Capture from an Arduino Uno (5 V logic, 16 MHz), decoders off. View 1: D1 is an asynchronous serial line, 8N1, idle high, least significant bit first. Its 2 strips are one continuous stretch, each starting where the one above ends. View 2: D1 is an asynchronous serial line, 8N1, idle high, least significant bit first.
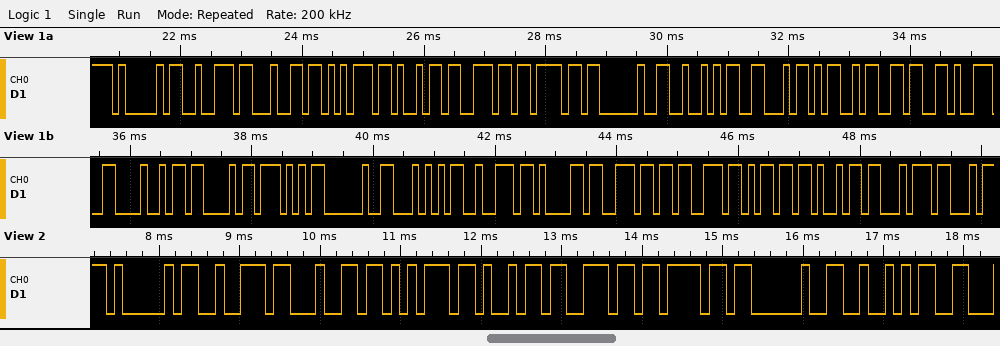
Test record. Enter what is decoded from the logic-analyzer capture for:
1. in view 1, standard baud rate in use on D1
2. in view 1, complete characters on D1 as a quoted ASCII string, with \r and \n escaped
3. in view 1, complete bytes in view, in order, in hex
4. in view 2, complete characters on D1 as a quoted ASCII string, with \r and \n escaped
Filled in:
9600 baud
"Arduino RFM69HCW Transmit"
0x41 0x72 0x64 0x75 0x69 0x6E 0x6F 0x20 0x52 0x46 0x4D 0x36 0x39 0x48 0x43 0x57 0x20 0x54 0x72 0x61 0x6E 0x73 0x6D 0x69 0x74
"Arduino R"
